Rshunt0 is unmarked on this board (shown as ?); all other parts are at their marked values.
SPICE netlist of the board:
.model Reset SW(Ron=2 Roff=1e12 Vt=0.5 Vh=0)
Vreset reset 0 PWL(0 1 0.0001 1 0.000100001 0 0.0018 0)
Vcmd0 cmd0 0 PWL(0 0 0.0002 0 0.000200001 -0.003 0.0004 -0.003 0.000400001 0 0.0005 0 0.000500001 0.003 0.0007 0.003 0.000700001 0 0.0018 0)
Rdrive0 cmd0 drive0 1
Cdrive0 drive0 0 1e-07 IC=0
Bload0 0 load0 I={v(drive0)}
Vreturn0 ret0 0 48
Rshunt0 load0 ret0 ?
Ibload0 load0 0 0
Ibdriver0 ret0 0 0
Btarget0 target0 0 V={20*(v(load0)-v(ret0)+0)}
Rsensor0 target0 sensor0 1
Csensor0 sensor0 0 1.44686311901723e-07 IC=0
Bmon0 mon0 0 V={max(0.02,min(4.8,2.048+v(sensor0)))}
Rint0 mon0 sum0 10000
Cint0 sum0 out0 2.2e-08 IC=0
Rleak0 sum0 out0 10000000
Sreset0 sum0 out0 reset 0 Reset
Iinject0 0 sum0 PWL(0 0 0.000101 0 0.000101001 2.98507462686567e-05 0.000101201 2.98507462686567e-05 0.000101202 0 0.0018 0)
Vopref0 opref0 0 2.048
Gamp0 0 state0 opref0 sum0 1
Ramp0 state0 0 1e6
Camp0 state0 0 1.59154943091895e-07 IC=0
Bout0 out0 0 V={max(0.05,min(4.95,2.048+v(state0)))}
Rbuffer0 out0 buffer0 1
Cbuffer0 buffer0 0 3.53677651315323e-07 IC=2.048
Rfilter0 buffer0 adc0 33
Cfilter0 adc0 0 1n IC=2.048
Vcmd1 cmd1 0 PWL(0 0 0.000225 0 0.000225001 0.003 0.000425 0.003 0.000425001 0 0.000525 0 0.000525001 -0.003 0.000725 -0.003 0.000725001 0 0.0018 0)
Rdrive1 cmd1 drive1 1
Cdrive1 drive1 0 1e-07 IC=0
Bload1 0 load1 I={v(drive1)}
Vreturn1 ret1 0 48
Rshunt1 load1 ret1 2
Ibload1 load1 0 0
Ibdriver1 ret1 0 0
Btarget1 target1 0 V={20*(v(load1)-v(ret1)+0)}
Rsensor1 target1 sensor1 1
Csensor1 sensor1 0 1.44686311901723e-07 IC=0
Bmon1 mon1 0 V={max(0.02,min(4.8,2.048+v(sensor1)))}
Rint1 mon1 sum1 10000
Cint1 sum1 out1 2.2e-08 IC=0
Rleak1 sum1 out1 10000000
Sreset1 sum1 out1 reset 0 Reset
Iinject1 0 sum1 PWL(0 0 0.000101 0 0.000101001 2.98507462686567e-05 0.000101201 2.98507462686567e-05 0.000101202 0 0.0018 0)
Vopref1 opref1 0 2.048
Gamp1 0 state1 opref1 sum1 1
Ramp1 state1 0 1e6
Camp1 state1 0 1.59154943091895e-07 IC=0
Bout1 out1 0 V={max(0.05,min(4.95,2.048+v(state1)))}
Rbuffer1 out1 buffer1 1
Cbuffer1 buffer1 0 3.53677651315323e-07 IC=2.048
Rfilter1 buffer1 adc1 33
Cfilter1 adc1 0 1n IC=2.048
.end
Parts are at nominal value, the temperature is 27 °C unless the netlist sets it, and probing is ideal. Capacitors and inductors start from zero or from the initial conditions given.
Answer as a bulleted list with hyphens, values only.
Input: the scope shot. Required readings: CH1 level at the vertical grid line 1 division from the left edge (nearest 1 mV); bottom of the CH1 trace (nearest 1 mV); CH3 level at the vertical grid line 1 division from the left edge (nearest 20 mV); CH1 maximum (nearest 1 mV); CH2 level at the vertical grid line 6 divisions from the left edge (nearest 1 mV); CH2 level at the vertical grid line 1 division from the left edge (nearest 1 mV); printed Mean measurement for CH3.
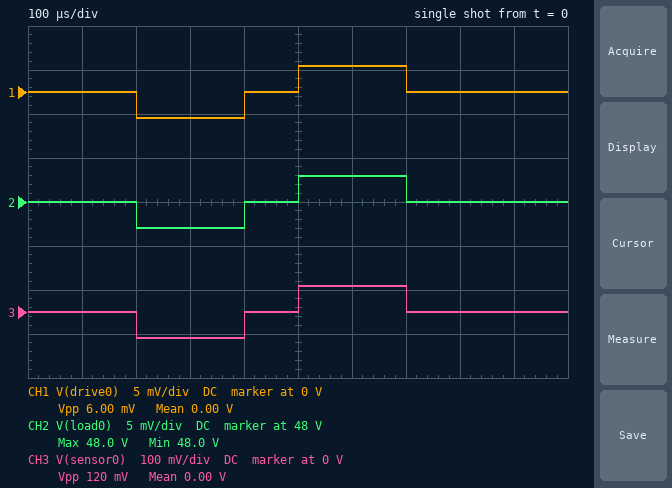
- 0 V
- -3 mV
- 0 V
- 3 mV
- 48.003 V
- 48.000 V
- 0.00 V
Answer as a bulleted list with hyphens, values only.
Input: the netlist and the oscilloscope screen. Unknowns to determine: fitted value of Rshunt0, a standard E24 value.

- 1 Ω
